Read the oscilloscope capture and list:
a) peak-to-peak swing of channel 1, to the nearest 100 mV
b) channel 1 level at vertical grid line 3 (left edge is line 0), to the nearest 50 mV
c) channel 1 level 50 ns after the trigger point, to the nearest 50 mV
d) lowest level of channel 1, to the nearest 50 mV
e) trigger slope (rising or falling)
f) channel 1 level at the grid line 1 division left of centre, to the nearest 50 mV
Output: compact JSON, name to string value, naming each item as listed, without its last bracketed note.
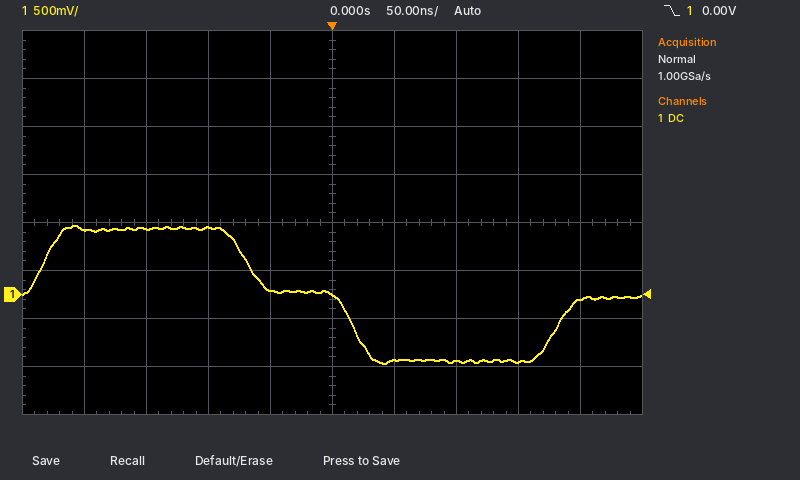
{"peak-to-peak swing of channel 1, to the nearest 100 mV": "1.40 V", "channel 1 level at vertical grid line 3 (left edge is line 0), to the nearest 50 mV": "700 mV", "channel 1 level 50 ns after the trigger point, to the nearest 50 mV": "-700 mV", "lowest level of channel 1, to the nearest 50 mV": "-700 mV", "trigger slope": "falling", "channel 1 level at the grid line 1 division left of centre, to the nearest 50 mV": "50 mV"}
